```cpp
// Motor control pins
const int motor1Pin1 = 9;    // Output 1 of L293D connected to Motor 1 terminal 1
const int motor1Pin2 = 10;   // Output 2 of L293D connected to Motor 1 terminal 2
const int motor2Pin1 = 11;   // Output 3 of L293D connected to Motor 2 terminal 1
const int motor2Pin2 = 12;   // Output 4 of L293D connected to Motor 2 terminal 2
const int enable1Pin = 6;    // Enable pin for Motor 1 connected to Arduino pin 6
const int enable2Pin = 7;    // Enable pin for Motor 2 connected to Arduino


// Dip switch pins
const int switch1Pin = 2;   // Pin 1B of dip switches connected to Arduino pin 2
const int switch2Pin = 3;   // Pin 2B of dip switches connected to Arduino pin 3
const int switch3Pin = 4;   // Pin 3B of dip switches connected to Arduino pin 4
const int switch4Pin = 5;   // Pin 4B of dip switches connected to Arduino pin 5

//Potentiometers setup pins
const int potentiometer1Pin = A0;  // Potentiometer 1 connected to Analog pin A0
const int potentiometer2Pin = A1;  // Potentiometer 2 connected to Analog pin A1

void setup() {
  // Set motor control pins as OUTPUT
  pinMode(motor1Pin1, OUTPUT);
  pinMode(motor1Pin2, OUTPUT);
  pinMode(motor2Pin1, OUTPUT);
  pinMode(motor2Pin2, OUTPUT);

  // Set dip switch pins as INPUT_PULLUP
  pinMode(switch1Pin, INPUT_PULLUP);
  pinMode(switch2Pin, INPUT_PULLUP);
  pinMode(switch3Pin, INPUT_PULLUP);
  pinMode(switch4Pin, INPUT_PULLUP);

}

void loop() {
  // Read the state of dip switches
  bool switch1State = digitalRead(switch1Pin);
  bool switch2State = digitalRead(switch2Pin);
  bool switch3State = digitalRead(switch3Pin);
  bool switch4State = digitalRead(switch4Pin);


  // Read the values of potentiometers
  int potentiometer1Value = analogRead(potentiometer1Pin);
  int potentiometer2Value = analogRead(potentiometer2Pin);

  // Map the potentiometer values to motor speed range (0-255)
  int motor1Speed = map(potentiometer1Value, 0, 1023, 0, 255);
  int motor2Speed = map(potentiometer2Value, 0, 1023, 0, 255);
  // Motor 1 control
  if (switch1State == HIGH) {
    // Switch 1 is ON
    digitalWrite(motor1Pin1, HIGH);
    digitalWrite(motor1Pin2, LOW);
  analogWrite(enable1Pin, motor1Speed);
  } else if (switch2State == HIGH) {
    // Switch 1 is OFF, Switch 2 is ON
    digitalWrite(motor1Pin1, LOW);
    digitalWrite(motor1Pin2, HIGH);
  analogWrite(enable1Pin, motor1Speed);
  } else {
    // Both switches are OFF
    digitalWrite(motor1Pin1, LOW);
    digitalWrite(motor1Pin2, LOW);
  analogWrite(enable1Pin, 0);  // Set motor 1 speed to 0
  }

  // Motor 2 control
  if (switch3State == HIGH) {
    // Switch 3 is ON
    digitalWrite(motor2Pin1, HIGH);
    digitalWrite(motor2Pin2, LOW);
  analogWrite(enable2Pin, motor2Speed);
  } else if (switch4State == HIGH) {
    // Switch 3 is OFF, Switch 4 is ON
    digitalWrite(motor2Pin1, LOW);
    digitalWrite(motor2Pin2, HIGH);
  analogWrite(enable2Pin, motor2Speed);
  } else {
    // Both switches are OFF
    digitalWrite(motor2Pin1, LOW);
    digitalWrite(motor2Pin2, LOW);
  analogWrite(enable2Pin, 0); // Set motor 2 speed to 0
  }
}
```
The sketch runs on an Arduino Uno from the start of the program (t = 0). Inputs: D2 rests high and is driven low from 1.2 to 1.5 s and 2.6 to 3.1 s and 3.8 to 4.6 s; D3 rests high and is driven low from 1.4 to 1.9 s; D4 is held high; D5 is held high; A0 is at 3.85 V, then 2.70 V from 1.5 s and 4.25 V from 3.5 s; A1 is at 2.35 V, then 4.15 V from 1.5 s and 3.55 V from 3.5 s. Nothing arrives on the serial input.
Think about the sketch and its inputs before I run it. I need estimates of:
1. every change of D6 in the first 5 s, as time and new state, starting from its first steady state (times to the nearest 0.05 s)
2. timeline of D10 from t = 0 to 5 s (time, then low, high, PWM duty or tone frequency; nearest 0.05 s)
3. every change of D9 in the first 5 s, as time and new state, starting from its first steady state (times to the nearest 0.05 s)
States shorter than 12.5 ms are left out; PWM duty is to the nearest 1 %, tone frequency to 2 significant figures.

0 s PWM 77 %; 1.4 s low; 1.5 s PWM 54 %; 3.5 s PWM 85 %
0 s low; 1.2 s high; 1.4 s low; 2.6 s high; 3.1 s low; 3.8 s high; 4.6 s low
0 s high; 1.2 s low; 1.5 s high; 2.6 s low; 3.1 s high; 3.8 s low; 4.6 s high
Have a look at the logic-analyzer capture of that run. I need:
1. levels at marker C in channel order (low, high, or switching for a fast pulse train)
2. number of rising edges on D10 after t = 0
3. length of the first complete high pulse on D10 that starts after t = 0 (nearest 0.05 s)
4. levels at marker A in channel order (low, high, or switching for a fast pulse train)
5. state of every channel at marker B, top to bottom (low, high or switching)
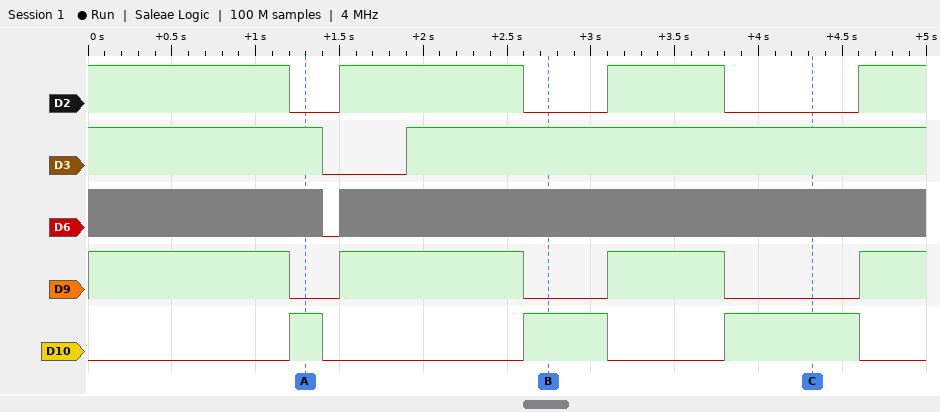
D2 low, D3 high, D6 switching, D9 low, D10 high
3
0.20 s
D2 low, D3 high, D6 switching, D9 low, D10 high
D2 low, D3 high, D6 switching, D9 low, D10 high
